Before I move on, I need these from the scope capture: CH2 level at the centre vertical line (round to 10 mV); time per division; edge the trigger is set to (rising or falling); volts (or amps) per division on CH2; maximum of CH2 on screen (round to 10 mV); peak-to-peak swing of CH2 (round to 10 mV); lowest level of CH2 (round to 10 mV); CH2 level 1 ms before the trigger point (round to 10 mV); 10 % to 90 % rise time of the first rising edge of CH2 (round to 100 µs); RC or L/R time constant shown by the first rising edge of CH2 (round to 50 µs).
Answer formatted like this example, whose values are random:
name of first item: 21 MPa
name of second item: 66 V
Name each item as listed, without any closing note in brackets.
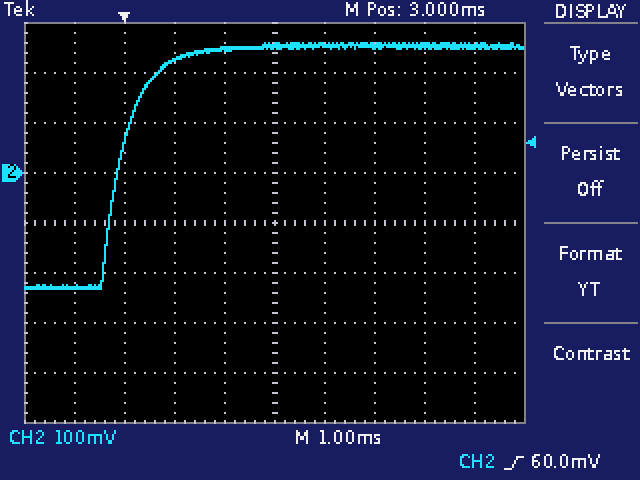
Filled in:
CH2 level at the centre vertical line: 250 mV
time per division: 1 ms
edge the trigger is set to: rising
volts (or amps) per division on CH2: 100 mV
maximum of CH2 on screen: 260 mV
peak-to-peak swing of CH2: 490 mV
lowest level of CH2: -230 mV
CH2 level 1 ms before the trigger point: -230 mV
10 % to 90 % rise time of the first rising edge of CH2: 1.1 ms
RC or L/R time constant shown by the first rising edge of CH2: 500 µs
